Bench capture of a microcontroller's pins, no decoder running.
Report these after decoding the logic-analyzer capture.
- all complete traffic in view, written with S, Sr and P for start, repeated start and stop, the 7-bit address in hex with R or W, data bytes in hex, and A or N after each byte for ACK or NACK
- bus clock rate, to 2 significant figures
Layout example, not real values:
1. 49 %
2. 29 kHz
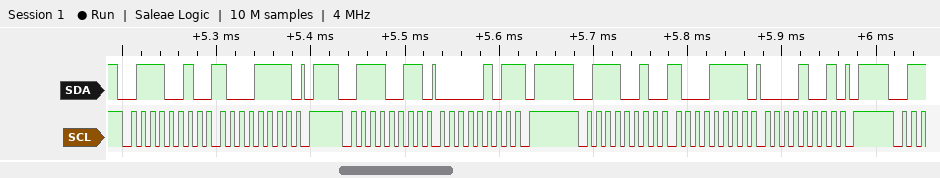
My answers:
1. S 39W A 8F A P S 39R A 05 N P S 39W A 8F A 09 A P
2. 100 kHz
